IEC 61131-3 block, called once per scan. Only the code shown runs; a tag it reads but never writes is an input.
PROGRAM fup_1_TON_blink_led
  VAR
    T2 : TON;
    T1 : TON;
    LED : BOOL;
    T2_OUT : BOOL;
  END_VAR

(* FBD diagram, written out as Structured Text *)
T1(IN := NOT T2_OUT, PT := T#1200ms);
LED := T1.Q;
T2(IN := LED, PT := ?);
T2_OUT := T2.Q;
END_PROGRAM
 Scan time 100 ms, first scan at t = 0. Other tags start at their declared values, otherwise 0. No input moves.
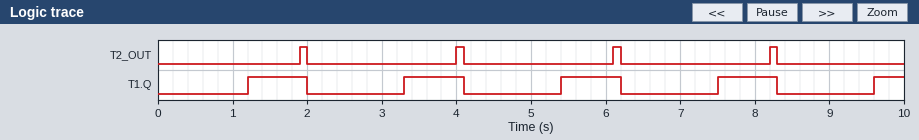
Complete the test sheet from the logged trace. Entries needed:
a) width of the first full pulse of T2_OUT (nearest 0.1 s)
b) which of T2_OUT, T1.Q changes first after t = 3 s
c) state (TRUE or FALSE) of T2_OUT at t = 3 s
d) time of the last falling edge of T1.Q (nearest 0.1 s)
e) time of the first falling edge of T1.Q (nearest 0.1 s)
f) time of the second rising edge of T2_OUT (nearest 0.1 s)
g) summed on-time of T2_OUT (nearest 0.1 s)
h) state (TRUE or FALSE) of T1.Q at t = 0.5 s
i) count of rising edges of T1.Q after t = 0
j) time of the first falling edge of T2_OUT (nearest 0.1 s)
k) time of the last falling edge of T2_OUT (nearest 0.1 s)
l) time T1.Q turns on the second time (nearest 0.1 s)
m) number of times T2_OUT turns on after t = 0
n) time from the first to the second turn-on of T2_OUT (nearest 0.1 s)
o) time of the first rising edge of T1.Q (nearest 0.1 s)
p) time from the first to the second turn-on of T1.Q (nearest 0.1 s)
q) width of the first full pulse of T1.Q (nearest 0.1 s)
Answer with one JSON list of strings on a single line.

["0.1 s", "T1.Q", "FALSE", "8.3 s", "2.0 s", "4.0 s", "0.4 s", "FALSE", "5", "2.0 s", "8.3 s", "3.3 s", "4", "2.1 s", "1.2 s", "2.1 s", "0.8 s"]
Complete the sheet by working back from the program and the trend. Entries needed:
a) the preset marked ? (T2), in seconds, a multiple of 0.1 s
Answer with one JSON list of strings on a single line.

["0.7 s"]
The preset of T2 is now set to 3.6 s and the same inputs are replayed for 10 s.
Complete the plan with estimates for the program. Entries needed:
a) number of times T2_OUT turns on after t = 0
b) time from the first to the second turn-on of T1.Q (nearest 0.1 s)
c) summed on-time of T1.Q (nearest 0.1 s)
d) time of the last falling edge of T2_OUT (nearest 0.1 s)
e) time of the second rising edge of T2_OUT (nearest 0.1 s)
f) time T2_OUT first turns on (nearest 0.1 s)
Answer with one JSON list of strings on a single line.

["2", "5.0 s", "7.4 s", "9.9 s", "9.8 s", "4.8 s"]
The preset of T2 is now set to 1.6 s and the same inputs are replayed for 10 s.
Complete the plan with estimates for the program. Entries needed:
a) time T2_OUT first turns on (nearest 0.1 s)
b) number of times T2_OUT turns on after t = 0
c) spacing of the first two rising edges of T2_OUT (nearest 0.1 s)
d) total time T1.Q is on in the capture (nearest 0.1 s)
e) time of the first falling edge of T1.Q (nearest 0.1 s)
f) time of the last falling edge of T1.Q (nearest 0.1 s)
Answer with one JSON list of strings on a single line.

["2.8 s", "3", "3.0 s", "5.1 s", "2.9 s", "8.9 s"]
